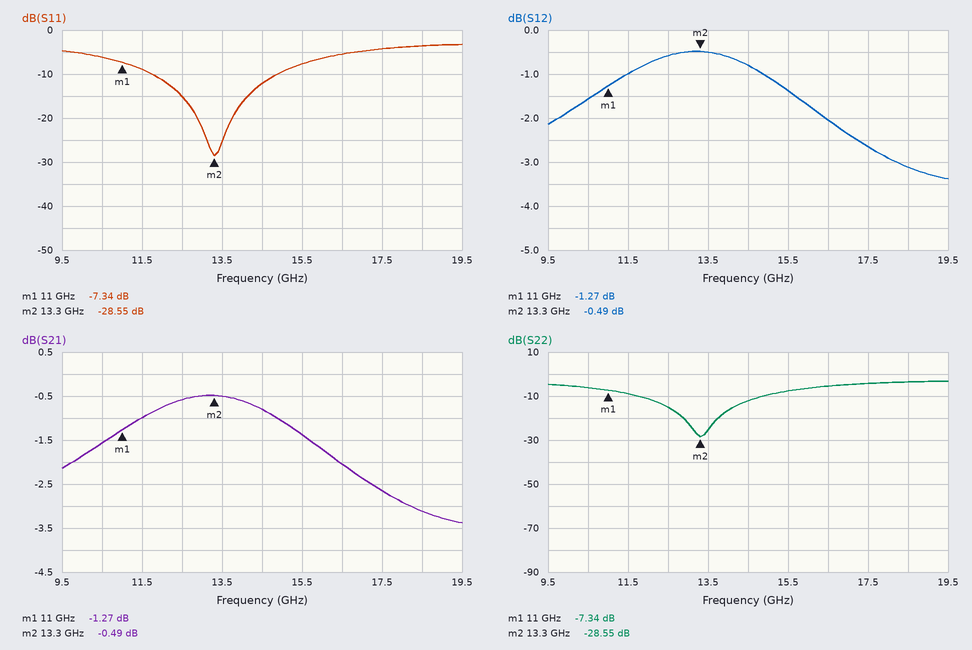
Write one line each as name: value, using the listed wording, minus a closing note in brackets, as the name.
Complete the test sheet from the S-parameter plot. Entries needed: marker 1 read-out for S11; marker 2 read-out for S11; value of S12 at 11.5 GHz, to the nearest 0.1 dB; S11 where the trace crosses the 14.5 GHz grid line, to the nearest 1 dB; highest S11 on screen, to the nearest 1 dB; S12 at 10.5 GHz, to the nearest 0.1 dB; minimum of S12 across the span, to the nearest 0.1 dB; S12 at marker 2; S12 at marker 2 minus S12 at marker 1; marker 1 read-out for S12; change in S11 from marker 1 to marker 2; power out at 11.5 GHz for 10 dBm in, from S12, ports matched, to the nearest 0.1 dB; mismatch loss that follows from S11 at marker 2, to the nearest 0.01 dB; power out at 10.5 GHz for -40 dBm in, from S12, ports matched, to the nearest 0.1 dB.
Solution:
marker 1 read-out for S11: -7.34 dB
marker 2 read-out for S11: -28.55 dB
value of S12 at 11.5 GHz, to the nearest 0.1 dB: -1.0 dB
S11 where the trace crosses the 14.5 GHz grid line, to the nearest 1 dB: -12 dB
highest S11 on screen, to the nearest 1 dB: -3 dB
S12 at 10.5 GHz, to the nearest 0.1 dB: -1.6 dB
minimum of S12 across the span, to the nearest 0.1 dB: -3.4 dB
S12 at marker 2: -0.49 dB
S12 at marker 2 minus S12 at marker 1: 0.78 dB
marker 1 read-out for S12: -1.27 dB
change in S11 from marker 1 to marker 2: -21.21 dB
power out at 11.5 GHz for 10 dBm in, from S12, ports matched, to the nearest 0.1 dB: 9.0 dBm
mismatch loss that follows from S11 at marker 2, to the nearest 0.01 dB: 0.01 dB
power out at 10.5 GHz for -40 dBm in, from S12, ports matched, to the nearest 0.1 dB: -41.6 dBm
